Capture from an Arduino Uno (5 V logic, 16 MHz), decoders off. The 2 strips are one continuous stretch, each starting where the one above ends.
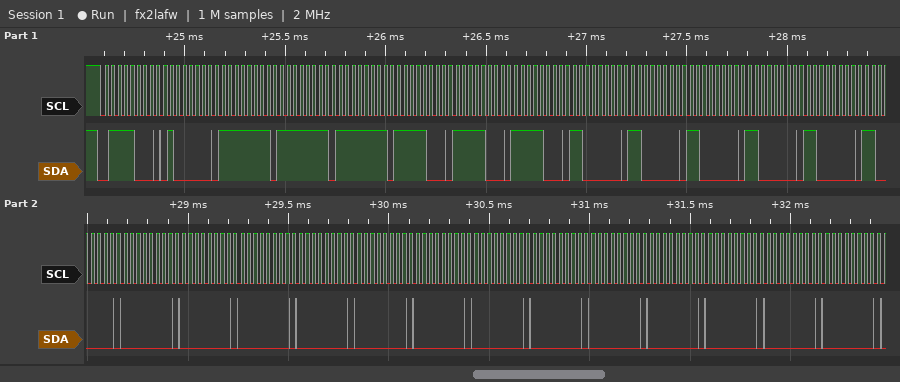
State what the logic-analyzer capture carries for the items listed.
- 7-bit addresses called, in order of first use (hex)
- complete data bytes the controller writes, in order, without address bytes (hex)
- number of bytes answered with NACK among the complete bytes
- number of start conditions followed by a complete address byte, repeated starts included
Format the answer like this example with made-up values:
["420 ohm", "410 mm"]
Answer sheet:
["0x3C", "40 FF FF FF F8 F8 F8 C0 C0 C0 C0 C0 C0 00 00 00 00 00 00 00 00 00 00 00 00 00", "0", "1"]
